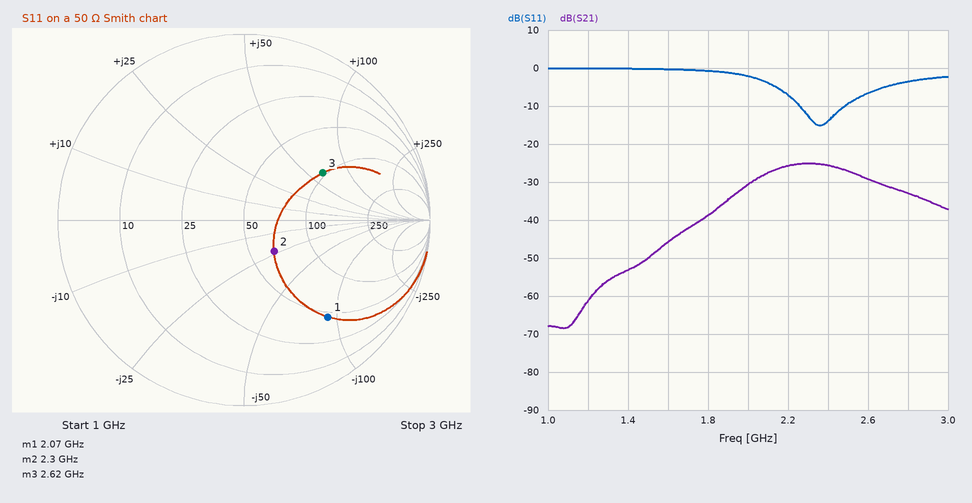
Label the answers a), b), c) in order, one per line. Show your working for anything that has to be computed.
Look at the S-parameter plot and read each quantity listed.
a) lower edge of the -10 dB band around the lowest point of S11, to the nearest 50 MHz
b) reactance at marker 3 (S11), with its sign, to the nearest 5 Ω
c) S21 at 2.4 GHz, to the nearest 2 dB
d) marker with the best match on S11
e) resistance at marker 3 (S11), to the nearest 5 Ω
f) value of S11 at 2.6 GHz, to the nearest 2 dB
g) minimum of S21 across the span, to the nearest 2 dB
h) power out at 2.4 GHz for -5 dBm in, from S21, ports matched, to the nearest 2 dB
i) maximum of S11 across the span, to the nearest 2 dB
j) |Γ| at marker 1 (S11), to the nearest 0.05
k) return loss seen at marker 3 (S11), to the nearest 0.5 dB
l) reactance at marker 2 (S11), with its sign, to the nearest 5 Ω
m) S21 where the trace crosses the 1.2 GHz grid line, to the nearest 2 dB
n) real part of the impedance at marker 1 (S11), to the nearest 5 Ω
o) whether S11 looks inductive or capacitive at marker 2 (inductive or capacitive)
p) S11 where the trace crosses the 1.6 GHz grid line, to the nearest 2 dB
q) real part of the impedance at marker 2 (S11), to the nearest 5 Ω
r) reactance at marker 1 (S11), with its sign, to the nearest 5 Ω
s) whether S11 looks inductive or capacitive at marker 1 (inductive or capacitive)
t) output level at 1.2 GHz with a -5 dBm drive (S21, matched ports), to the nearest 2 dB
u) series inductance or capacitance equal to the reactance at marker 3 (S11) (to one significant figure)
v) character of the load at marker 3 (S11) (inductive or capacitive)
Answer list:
a) 2.25 GHz
b) +65 Ω
c) -26 dB
d) marker 2
e) 95 Ω
f) -6 dB
g) -68 dB
h) -5 dBm + (-26 dB) = -30 dBm
i) 0 dB
j) 0.70
k) 6.0 dB
l) -25 Ω
m) -62 dB
n) 45 Ω
o) capacitive
p) 0 dB
q) 65 Ω
r) -90 Ω
s) capacitive
t) -5 dBm + (-62 dB) = -66 dBm
u) L = 65 Ω/(2π × 2.62 GHz) ≈ 4 nH
v) inductive
